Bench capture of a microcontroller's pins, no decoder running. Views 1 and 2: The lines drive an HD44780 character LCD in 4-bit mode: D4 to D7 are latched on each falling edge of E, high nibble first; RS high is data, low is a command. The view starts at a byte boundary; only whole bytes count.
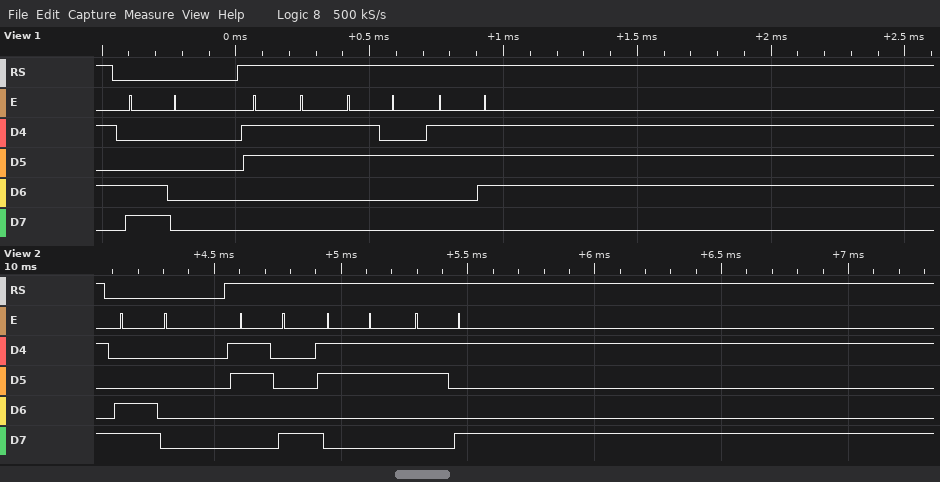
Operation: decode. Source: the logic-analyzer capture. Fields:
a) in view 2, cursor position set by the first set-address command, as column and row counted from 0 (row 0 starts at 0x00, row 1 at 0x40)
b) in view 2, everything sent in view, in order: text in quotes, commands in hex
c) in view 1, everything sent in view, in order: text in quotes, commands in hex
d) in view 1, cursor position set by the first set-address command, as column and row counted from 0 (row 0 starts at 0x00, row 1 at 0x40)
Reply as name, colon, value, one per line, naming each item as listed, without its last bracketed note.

in view 2, cursor position set by the first set-address command, as column and row counted from 0: column 0, row 1
in view 2, everything sent in view, in order: text in quotes, commands in hex: 0xC0 "839"
in view 1, everything sent in view, in order: text in quotes, commands in hex: 0xC0 "327"
in view 1, cursor position set by the first set-address command, as column and row counted from 0: column 0, row 1
